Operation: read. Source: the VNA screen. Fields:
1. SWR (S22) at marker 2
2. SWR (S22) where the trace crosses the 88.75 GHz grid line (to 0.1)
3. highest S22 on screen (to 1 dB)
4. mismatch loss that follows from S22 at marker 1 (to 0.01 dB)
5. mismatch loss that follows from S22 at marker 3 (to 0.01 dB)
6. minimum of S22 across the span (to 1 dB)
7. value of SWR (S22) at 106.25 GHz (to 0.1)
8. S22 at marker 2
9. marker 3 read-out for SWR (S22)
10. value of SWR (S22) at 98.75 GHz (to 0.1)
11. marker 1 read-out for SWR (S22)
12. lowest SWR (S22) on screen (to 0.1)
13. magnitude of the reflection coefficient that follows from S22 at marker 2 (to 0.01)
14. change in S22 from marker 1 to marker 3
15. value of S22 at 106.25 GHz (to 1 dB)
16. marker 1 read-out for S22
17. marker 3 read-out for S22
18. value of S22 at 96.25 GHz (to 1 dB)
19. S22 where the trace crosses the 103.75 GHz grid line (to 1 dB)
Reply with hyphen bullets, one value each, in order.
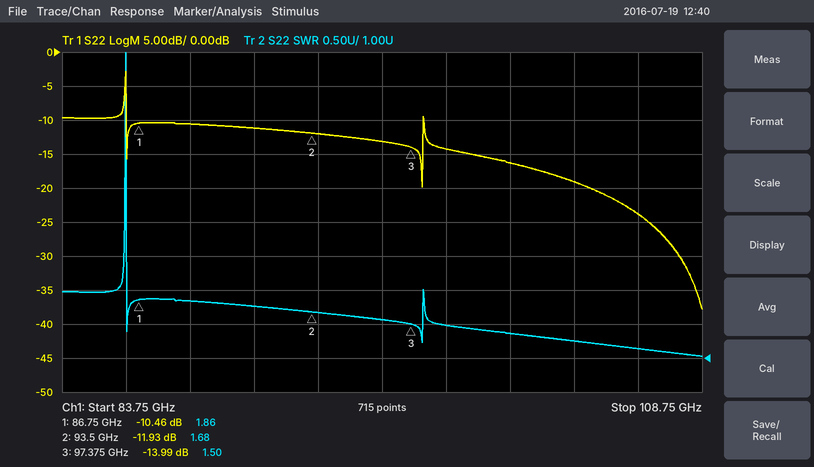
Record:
- 1.68
- 1.8
- -3 dB
- 0.41 dB
- 0.18 dB
- -38 dB
- 1.1
- -11.93 dB
- 1.50
- 1.5
- 1.86
- 1.0
- 0.25
- -3.53 dB
- -24 dB
- -10.46 dB
- -13.99 dB
- -13 dB
- -19 dB
